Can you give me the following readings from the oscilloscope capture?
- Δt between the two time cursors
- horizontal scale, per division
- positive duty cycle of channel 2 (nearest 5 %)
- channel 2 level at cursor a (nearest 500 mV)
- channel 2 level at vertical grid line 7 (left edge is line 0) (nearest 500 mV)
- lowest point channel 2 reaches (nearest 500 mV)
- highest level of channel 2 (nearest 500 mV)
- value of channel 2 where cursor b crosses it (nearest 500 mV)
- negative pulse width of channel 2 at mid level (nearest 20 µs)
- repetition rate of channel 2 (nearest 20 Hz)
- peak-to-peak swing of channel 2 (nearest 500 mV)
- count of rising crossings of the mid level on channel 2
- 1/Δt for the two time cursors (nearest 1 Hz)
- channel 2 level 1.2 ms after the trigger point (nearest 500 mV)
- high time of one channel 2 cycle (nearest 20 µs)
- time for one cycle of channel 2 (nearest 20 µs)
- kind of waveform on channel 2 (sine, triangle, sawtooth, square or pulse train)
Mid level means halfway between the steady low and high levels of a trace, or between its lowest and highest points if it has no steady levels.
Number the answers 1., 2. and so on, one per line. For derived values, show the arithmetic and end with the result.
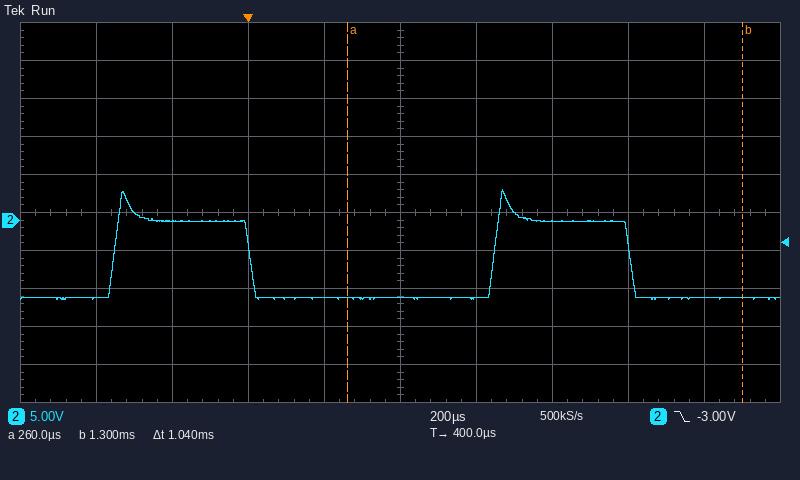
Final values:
1. 1.04 ms
2. 200 µs
3. 360 µs / 1.00 ms ≈ 36.0 %, so 35 % to the nearest 5 %
4. -10.0 V
5. 0.0 V
6. -10.5 V
7. 4.0 V
8. -10.0 V
9. 640 µs
10. 1 / 1.00 ms ≈ 1.00 kHz
11. 4.0 V − (-10.5 V) = 14.5 V
12. 2
13. 1 / 1.04 ms ≈ 962 Hz
14. -10.0 V
15. 360 µs
16. 1.00 ms
17. pulse train
